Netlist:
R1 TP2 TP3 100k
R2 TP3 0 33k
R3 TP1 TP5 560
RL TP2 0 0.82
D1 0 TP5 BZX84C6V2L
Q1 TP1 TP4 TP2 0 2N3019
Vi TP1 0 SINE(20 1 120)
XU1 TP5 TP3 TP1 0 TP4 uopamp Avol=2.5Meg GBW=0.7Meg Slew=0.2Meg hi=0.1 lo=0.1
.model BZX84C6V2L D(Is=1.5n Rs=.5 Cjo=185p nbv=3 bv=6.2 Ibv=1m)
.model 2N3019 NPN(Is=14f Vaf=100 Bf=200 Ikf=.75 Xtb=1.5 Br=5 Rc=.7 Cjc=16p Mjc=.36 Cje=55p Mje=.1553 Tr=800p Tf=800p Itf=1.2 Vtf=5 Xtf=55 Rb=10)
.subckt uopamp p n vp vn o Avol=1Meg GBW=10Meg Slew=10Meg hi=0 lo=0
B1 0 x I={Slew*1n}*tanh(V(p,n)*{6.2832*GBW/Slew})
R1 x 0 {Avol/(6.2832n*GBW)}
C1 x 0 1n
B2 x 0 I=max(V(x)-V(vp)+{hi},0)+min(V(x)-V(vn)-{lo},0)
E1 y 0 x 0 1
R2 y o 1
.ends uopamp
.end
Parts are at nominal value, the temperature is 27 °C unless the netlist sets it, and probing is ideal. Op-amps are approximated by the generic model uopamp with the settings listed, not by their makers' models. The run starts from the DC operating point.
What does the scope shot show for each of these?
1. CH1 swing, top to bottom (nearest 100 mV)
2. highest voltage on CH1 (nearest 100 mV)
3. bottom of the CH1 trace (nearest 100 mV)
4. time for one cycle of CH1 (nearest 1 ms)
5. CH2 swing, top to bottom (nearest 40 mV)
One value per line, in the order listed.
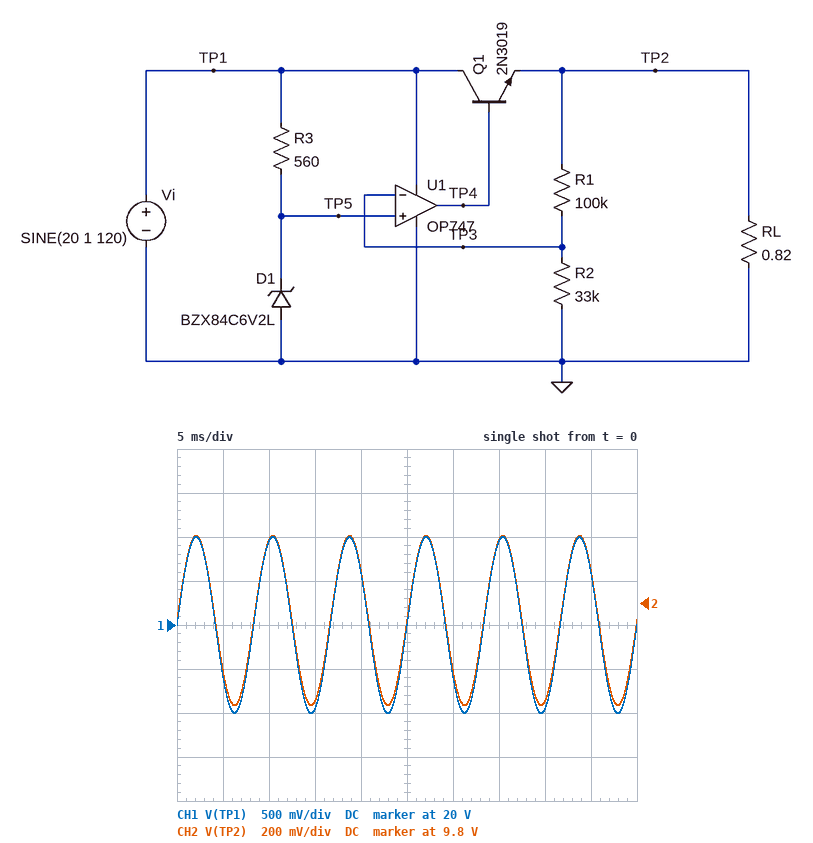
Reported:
2.0 V
21.0 V
19.0 V
8 ms
760 mV
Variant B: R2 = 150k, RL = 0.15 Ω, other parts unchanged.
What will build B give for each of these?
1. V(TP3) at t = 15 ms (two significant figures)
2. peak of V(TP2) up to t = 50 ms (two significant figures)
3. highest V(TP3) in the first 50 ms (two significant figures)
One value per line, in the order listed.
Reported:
1.5 V
2.6 V
1.6 V
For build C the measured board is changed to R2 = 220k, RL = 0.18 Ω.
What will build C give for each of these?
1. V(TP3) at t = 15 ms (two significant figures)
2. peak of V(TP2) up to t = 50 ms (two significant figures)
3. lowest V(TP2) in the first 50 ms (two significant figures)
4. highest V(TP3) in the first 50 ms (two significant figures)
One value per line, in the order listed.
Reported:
2.0 V
3.1 V
2.9 V
2.1 V
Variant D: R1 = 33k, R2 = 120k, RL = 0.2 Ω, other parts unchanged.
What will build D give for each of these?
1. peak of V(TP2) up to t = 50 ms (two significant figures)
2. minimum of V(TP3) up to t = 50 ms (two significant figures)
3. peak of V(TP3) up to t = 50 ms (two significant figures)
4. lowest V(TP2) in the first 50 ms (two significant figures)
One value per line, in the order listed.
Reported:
3.4 V
2.5 V
2.7 V
3.2 V
